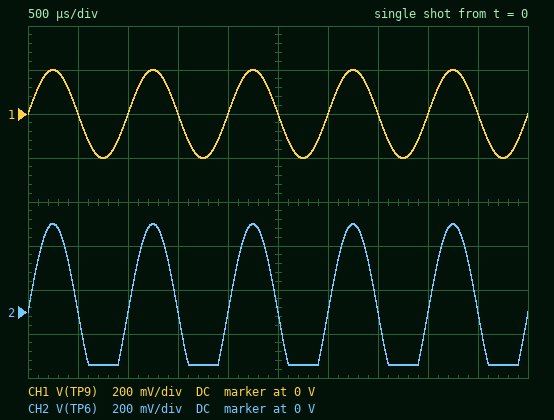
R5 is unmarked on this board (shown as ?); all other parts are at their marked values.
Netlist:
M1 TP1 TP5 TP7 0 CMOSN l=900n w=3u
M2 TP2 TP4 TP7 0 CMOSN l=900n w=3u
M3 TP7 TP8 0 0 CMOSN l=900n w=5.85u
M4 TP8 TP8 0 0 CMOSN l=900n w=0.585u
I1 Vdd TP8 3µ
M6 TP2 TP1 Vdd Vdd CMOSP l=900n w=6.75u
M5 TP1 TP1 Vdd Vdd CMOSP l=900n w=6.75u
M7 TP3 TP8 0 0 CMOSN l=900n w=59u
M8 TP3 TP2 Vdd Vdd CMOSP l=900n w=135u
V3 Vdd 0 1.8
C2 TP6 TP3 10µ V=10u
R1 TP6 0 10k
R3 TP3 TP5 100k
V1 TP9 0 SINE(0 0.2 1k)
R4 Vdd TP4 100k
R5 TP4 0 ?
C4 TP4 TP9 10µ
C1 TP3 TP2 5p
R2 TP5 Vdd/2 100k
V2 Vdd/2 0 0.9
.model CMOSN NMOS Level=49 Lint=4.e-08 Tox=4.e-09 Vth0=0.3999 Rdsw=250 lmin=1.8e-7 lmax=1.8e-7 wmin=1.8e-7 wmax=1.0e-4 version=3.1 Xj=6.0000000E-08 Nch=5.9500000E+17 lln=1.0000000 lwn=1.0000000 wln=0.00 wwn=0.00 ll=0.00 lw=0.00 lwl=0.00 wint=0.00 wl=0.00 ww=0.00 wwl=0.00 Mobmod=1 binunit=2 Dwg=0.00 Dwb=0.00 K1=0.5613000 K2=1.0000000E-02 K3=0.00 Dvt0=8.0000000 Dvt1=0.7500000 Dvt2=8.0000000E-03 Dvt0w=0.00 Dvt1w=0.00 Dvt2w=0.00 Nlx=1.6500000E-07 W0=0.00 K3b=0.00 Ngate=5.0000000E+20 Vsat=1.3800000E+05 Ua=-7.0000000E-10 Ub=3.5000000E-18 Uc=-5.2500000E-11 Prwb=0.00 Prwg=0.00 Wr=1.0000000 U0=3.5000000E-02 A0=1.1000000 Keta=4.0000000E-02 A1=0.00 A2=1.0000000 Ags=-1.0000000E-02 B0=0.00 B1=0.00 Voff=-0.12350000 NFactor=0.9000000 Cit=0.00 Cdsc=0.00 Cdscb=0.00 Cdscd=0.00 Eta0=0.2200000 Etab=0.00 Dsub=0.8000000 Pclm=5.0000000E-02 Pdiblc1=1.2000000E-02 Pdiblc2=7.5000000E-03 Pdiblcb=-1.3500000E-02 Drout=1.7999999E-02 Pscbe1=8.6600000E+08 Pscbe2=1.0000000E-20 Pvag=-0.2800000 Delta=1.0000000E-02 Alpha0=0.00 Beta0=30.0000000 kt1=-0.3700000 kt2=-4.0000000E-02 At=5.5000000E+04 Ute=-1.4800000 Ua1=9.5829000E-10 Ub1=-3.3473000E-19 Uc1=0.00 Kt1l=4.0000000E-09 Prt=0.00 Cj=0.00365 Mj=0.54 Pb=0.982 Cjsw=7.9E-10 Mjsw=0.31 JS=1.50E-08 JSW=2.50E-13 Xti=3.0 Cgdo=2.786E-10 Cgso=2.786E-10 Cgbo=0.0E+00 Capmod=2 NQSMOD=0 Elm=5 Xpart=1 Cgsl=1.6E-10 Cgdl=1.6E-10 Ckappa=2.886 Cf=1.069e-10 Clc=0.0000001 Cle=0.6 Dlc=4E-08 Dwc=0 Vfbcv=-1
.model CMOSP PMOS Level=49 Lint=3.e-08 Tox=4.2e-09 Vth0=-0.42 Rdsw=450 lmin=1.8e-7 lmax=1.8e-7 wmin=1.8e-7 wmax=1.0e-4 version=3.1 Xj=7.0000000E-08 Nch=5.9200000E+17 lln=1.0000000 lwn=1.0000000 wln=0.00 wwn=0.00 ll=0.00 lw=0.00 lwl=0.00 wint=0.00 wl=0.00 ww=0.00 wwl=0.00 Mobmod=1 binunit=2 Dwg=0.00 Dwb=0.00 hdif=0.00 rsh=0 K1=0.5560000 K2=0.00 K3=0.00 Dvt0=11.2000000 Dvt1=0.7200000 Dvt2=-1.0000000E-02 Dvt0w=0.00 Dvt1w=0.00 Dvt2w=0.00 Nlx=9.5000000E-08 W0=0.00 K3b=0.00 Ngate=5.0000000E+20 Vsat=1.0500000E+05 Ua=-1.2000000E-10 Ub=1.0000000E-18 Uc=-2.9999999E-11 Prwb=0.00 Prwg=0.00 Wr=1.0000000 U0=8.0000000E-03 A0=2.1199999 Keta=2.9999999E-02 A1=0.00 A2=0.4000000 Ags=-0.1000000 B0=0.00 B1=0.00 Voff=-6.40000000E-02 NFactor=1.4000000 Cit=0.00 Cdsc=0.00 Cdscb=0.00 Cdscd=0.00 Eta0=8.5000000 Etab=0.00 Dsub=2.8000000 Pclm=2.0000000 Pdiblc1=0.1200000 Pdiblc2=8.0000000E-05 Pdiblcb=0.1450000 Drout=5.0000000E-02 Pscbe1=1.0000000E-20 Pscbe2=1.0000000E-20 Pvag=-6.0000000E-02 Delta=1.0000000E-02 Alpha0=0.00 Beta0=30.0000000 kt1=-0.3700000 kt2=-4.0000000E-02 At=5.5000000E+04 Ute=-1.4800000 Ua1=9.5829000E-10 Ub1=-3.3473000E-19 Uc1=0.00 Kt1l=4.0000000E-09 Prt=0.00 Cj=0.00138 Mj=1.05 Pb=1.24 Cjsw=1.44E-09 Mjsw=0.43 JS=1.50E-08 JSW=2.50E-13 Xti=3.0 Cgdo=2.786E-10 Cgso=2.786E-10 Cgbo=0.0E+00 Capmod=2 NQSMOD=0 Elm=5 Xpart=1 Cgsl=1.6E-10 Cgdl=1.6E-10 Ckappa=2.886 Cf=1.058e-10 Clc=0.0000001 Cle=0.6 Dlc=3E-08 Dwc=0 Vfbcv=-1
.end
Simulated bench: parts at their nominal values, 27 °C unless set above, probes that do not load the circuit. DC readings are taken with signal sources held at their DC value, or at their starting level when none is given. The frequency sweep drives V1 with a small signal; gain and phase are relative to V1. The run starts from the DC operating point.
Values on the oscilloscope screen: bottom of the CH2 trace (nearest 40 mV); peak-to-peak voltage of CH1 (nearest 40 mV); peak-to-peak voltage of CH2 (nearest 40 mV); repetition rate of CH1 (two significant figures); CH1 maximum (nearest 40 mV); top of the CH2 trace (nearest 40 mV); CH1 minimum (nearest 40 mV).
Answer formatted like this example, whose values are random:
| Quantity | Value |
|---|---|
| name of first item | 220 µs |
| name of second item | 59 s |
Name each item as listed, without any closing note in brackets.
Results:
| Quantity | Value |
|---|---|
| bottom of the CH2 trace | -240 mV |
| peak-to-peak voltage of CH1 | 400 mV |
| peak-to-peak voltage of CH2 | 640 mV |
| repetition rate of CH1 | 1.0 kHz |
| CH1 maximum | 200 mV |
| top of the CH2 trace | 400 mV |
| CH1 minimum | -200 mV |
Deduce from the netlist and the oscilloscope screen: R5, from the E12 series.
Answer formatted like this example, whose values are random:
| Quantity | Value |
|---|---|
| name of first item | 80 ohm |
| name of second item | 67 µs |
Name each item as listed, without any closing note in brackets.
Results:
| Quantity | Value |
|---|---|
| R5, from the E12 series | 47 kΩ |
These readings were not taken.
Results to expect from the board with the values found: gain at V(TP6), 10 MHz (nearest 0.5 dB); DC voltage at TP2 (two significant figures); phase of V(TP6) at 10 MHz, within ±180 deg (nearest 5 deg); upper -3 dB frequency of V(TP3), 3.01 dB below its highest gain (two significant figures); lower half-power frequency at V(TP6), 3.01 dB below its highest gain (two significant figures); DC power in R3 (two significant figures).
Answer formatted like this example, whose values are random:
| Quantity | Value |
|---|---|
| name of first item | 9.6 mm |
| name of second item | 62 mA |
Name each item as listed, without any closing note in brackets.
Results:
| Quantity | Value |
|---|---|
| gain at V(TP6), 10 MHz | -13.5 dB |
| DC voltage at TP2 | 1.1 V |
| phase of V(TP6) at 10 MHz, within ±180 deg | -100 deg |
| upper -3 dB frequency of V(TP3), 3.01 dB below its highest gain | 1.1 MHz |
| lower half-power frequency at V(TP6), 3.01 dB below its highest gain | 1.7 Hz |
| DC power in R3 | 1.1 µW |
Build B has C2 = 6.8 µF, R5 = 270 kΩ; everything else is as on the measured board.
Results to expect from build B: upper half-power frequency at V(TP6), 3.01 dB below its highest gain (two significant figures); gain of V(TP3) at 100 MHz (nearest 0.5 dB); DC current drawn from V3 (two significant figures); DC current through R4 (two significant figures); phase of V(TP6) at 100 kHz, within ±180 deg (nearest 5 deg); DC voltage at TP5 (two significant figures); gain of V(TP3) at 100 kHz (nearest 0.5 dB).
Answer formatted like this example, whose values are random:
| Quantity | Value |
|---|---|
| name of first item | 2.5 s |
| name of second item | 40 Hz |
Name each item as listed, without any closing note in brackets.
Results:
| Quantity | Value |
|---|---|
| upper half-power frequency at V(TP6), 3.01 dB below its highest gain | 410 kHz |
| gain of V(TP3) at 100 MHz | -32.5 dB |
| DC current drawn from V3 | 380 µA |
| DC current through R4 | 4.9 µA |
| phase of V(TP6) at 100 kHz, within ±180 deg | -15 deg |
| DC voltage at TP5 | 1.3 V |
| gain of V(TP3) at 100 kHz | 3.5 dB |
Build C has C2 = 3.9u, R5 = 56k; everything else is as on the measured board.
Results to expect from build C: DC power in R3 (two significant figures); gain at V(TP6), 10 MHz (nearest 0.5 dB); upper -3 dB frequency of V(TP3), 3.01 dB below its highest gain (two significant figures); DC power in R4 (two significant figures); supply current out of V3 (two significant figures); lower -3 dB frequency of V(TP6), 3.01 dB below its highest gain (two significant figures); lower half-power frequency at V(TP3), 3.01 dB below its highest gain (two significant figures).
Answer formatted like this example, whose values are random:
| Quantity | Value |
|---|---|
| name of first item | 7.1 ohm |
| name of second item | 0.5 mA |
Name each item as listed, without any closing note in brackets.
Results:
| Quantity | Value |
|---|---|
| DC power in R3 | 650 nW |
| gain at V(TP6), 10 MHz | -10.5 dB |
| upper -3 dB frequency of V(TP3), 3.01 dB below its highest gain | 1.5 MHz |
| DC power in R4 | 13 µW |
| supply current out of V3 | 320 µA |
| lower -3 dB frequency of V(TP6), 3.01 dB below its highest gain | 4.1 Hz |
| lower half-power frequency at V(TP3), 3.01 dB below its highest gain | 440 mHz |
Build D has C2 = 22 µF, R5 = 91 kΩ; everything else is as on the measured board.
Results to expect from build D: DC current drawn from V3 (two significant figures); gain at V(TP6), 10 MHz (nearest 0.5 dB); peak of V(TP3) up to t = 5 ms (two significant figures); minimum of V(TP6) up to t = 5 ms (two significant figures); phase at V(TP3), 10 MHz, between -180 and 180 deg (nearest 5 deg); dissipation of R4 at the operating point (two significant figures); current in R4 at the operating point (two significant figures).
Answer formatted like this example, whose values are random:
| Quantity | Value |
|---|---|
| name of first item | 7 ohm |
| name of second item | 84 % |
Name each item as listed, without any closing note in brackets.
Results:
| Quantity | Value |
|---|---|
| DC current drawn from V3 | 350 µA |
| gain at V(TP6), 10 MHz | -8.5 dB |
| peak of V(TP3) up to t = 5 ms | 1.2 V |
| minimum of V(TP6) up to t = 5 ms | -400 mV |
| phase at V(TP3), 10 MHz, between -180 and 180 deg | -95 deg |
| dissipation of R4 at the operating point | 8.9 µW |
| current in R4 at the operating point | 9.4 µA |
